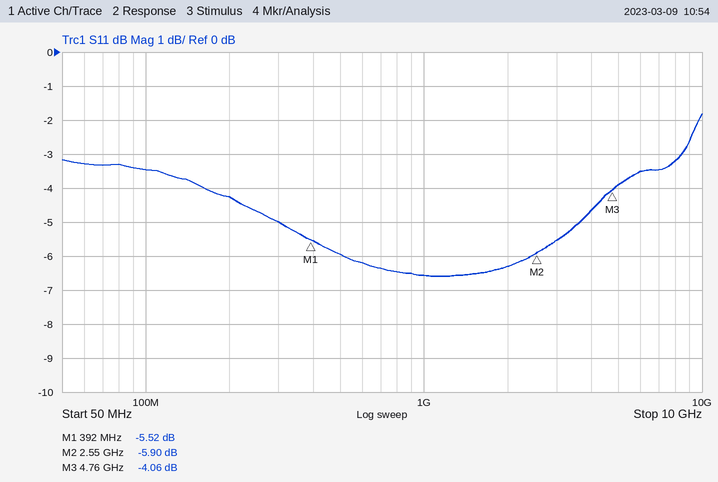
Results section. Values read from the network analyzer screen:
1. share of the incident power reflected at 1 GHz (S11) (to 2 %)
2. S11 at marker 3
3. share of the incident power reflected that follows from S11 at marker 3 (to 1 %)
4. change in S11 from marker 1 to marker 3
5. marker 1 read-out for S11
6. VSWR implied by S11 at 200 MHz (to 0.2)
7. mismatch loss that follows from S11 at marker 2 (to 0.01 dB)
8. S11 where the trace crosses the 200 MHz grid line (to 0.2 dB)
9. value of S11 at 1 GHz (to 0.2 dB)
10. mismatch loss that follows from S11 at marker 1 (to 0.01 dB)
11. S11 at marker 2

22 %
-4.06 dB
39 %
1.46 dB
-5.52 dB
4.2
1.29 dB
-4.2 dB
-6.6 dB
1.43 dB
-5.90 dB
